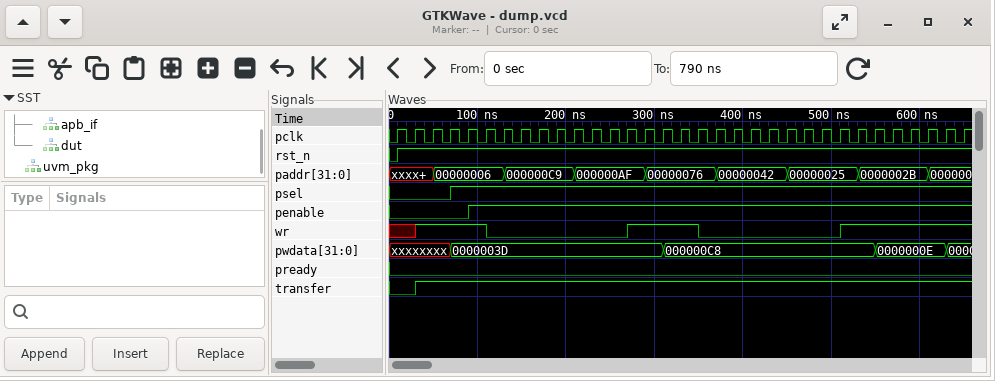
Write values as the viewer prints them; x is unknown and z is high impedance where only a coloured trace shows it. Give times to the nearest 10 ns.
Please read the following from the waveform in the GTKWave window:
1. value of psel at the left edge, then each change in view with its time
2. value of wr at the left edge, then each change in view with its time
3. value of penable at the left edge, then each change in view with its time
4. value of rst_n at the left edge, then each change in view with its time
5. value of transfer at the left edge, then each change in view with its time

0, 1 at 70 ns
x, 1 at 30 ns, 0 at 110 ns, 1 at 270 ns, 0 at 350 ns, 1 at 510 ns
0, 1 at 90 ns
0, 1 at 10 ns
0, 1 at 30 ns
